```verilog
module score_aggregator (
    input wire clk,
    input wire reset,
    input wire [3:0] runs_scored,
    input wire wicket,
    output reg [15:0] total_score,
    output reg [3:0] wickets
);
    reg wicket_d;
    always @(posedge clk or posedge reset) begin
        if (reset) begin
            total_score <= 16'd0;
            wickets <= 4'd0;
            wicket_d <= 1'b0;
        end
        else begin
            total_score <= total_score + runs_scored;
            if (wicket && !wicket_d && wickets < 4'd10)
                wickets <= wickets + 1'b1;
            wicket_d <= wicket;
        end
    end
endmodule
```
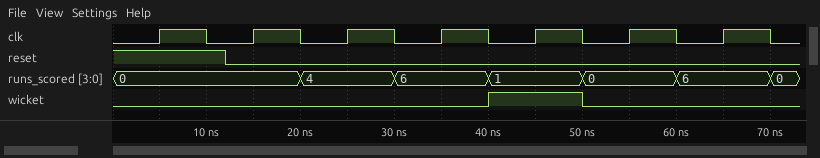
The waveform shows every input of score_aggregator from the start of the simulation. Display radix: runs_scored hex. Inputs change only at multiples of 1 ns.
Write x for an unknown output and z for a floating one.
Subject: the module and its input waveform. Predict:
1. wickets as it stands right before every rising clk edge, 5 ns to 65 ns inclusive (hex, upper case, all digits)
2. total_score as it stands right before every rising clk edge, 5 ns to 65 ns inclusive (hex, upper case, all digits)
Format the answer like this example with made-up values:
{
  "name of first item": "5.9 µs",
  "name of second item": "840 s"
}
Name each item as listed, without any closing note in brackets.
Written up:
{
  "wickets as it stands right before every rising clk edge, 5 ns to 65 ns inclusive": "0, 0, 0, 0, 0, 1, 1",
  "total_score as it stands right before every rising clk edge, 5 ns to 65 ns inclusive": "0000, 0000, 0000, 0004, 000A, 000B, 000B"
}
